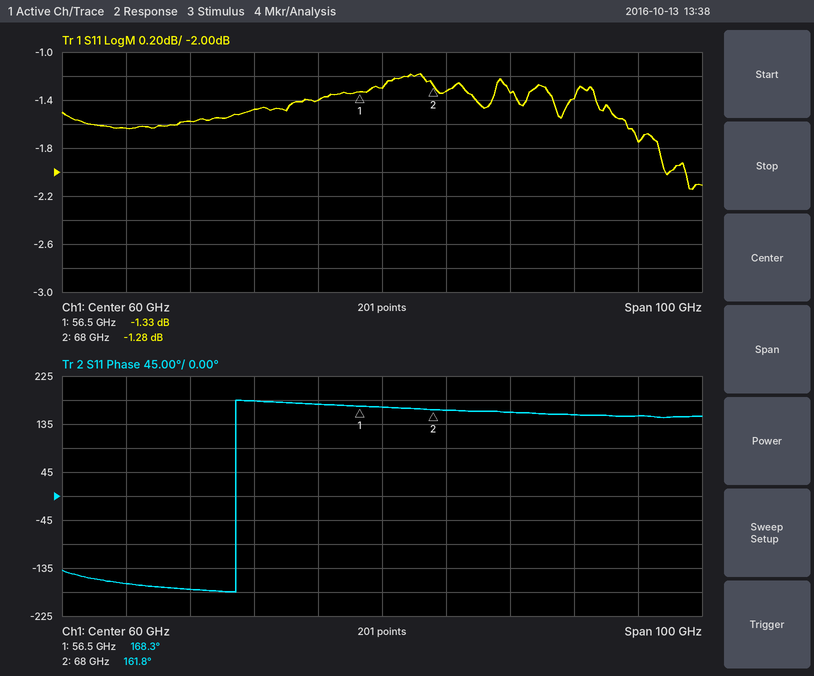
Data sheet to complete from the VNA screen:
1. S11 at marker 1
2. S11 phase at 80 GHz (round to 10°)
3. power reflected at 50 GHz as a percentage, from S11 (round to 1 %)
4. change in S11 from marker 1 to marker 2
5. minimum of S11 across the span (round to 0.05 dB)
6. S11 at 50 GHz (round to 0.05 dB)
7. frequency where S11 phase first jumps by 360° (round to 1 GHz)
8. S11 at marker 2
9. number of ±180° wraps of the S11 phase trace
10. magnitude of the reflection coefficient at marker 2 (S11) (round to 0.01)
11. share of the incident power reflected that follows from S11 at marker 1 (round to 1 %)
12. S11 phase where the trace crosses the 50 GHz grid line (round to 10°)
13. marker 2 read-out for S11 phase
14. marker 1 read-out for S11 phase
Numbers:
-1.33 dB
160°
72 %
0.05 dB
-2.15 dB
-1.40 dB
37 GHz
-1.28 dB
1
0.86
74 %
170°
161.8°
168.3°
